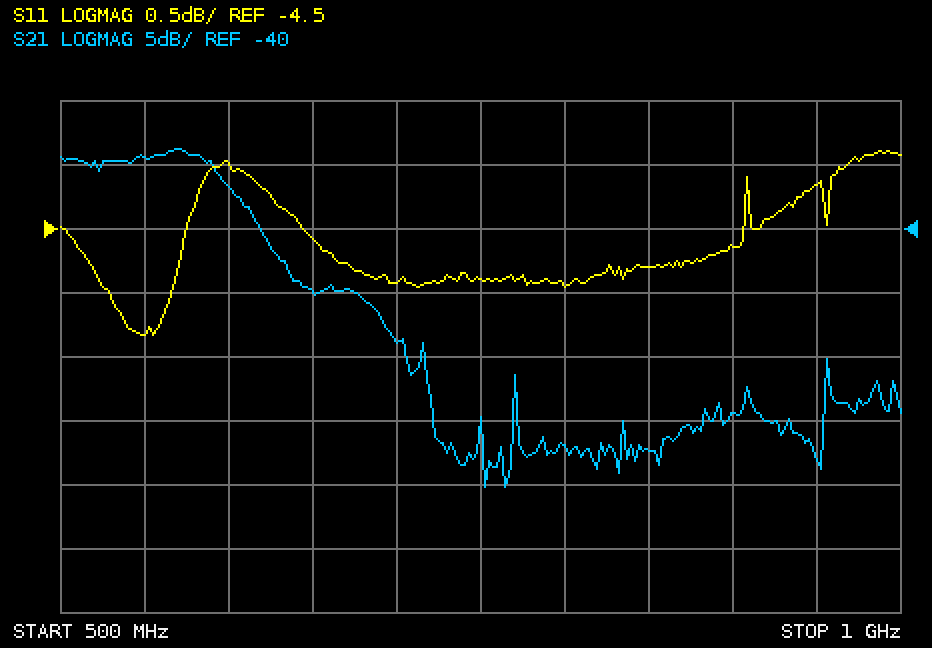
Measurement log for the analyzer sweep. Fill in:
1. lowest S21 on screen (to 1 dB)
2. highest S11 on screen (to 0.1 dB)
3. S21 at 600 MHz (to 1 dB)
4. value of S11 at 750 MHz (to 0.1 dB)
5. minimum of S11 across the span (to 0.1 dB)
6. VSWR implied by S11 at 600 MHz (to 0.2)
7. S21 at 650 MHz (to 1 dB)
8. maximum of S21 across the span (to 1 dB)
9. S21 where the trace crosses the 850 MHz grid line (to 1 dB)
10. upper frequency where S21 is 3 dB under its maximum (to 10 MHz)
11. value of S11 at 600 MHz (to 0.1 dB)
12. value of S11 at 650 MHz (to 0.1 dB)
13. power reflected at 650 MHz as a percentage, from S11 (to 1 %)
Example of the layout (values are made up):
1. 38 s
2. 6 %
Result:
1. -60 dB
2. -3.9 dB
3. -37 dB
4. -4.9 dB
5. -5.3 dB
6. 4.4
7. -45 dB
8. -34 dB
9. -57 dB
10. 600 MHz
11. -4.0 dB
12. -4.6 dB
13. 35 %
